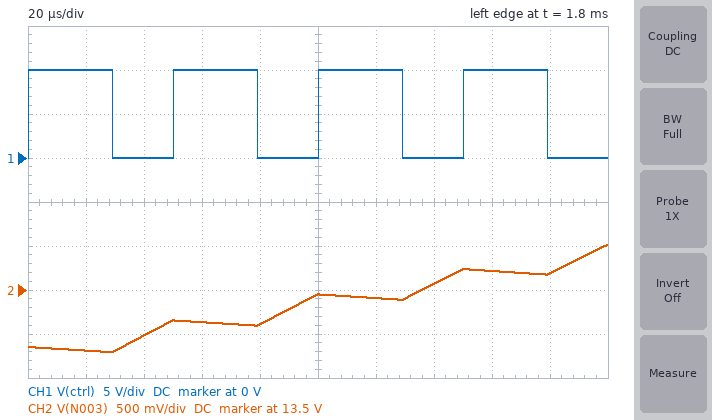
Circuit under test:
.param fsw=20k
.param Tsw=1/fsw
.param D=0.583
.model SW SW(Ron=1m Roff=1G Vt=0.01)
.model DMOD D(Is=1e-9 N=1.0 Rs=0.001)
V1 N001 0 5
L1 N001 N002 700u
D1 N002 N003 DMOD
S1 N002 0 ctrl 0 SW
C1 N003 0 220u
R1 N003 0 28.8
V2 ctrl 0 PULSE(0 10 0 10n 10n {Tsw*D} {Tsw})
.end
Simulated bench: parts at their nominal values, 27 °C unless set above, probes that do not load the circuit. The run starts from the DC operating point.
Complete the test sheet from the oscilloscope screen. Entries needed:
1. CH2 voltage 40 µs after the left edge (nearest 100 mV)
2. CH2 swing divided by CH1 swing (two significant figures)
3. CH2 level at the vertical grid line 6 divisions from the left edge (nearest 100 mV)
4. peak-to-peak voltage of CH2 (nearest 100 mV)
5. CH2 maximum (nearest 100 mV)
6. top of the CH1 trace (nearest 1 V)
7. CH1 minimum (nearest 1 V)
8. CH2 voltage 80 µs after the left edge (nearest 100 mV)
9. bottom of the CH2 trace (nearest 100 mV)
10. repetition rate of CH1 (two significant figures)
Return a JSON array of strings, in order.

["13.0 V", "0.12", "13.4 V", "1.2 V", "14.0 V", "10 V", "0 V", "13.1 V", "12.8 V", "20 kHz"]
